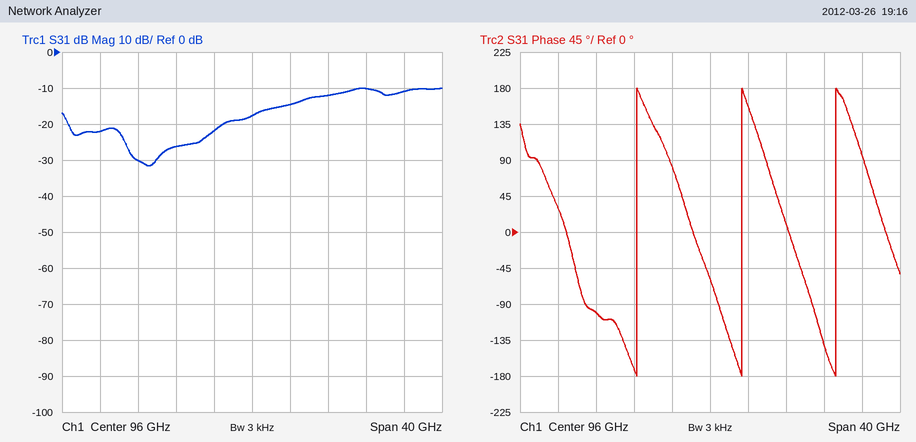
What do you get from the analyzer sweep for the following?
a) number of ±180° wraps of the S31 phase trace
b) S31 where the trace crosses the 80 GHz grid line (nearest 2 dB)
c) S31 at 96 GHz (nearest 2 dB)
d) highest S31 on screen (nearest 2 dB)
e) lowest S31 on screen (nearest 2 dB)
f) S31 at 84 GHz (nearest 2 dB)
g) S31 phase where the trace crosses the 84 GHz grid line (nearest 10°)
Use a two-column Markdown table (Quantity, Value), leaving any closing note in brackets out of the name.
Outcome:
| Quantity | Value |
|---|---|
| number of ±180° wraps of the S31 phase trace | 3 |
| S31 where the trace crosses the 80 GHz grid line | -22 dB |
| S31 at 96 GHz | -18 dB |
| highest S31 on screen | -10 dB |
| lowest S31 on screen | -32 dB |
| S31 at 84 GHz | -30 dB |
| S31 phase where the trace crosses the 84 GHz grid line | -100° |
